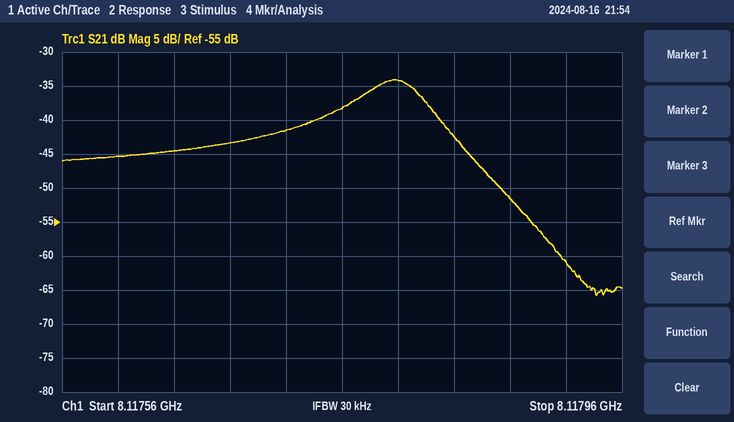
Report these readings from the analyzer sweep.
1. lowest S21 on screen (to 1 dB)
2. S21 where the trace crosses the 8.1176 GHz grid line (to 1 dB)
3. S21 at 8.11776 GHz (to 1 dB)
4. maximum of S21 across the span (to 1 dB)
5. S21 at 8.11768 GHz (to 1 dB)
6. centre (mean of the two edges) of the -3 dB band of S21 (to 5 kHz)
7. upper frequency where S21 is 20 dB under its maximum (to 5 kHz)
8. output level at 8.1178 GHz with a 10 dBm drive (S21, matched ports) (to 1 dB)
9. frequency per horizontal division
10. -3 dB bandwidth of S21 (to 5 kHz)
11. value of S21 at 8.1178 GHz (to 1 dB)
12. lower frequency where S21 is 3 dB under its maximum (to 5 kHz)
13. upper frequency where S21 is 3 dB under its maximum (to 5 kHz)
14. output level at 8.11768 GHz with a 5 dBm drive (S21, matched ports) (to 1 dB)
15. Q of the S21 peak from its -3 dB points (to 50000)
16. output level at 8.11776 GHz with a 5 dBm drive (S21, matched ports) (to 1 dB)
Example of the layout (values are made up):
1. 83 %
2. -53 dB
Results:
1. -66 dB
2. -45 dB
3. -38 dB
4. -34 dB
5. -43 dB
6. 8.117795 GHz
7. 8.117890 GHz
8. -24 dBm
9. 40 kHz
10. 50 kHz
11. -34 dB
12. 8.117770 GHz
13. 8.117820 GHz
14. -38 dBm
15. 150000
16. -33 dBm
